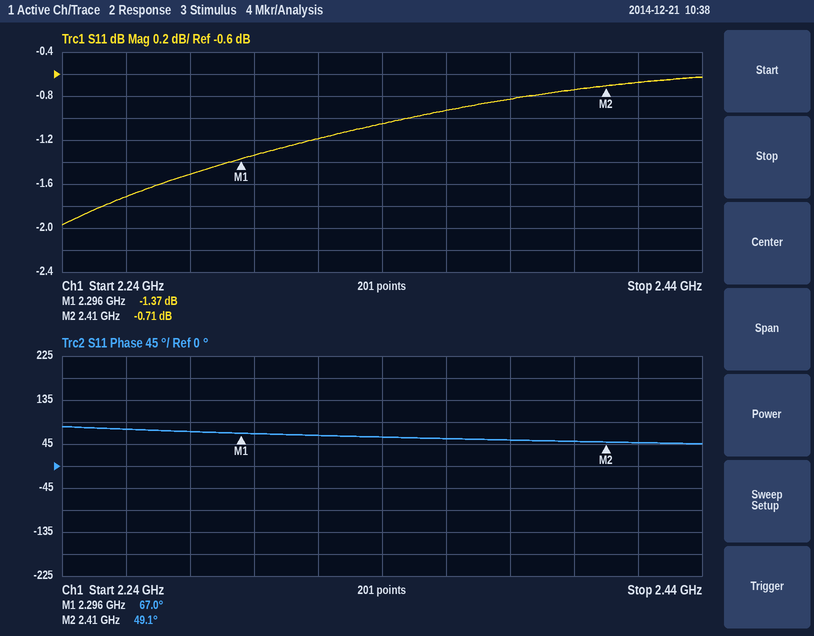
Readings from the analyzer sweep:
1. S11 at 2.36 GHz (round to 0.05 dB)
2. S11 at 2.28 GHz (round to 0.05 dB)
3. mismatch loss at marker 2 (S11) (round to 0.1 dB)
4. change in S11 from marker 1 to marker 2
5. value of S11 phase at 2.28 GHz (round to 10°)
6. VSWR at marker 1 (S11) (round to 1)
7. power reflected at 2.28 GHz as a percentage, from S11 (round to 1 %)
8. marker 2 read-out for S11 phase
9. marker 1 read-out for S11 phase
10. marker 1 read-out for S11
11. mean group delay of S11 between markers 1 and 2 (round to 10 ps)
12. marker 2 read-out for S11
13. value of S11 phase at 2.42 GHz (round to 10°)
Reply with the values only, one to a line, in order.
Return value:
-0.95 dB
-1.50 dB
8.2 dB
0.66 dB
70°
13
71 %
49.1°
67.0°
-1.37 dB
440 ps
-0.71 dB
50°
